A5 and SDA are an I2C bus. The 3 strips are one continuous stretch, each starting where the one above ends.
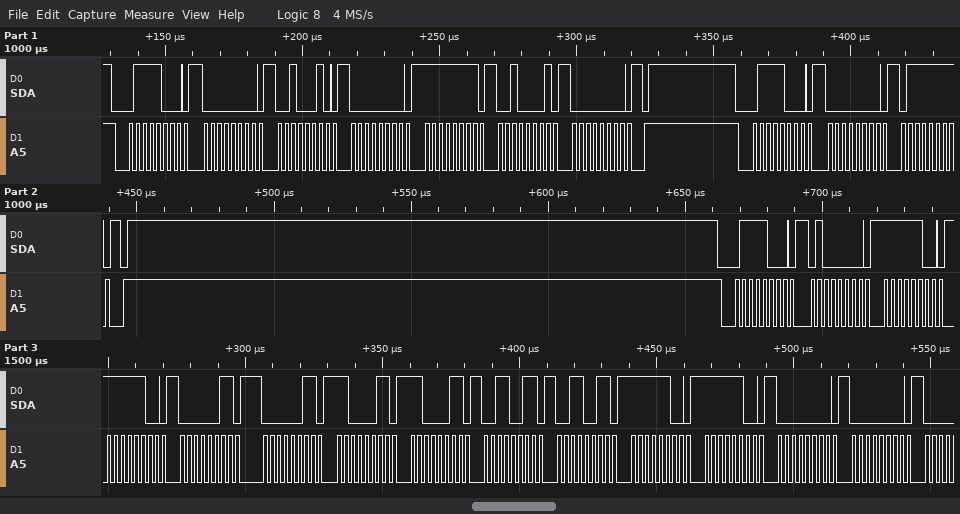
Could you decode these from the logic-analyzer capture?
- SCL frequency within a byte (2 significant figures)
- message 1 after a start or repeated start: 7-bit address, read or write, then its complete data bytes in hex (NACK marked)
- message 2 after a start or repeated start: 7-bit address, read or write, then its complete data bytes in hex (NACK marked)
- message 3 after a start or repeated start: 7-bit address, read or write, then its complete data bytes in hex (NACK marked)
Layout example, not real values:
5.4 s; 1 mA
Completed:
400 kHz; 0x3C write: 00 22 00 FF 21 00; 0x3C write: 00 7F; 0x3C write: 40 FC FC 03 03 C3 C3 33 33 FC FC 00 00
